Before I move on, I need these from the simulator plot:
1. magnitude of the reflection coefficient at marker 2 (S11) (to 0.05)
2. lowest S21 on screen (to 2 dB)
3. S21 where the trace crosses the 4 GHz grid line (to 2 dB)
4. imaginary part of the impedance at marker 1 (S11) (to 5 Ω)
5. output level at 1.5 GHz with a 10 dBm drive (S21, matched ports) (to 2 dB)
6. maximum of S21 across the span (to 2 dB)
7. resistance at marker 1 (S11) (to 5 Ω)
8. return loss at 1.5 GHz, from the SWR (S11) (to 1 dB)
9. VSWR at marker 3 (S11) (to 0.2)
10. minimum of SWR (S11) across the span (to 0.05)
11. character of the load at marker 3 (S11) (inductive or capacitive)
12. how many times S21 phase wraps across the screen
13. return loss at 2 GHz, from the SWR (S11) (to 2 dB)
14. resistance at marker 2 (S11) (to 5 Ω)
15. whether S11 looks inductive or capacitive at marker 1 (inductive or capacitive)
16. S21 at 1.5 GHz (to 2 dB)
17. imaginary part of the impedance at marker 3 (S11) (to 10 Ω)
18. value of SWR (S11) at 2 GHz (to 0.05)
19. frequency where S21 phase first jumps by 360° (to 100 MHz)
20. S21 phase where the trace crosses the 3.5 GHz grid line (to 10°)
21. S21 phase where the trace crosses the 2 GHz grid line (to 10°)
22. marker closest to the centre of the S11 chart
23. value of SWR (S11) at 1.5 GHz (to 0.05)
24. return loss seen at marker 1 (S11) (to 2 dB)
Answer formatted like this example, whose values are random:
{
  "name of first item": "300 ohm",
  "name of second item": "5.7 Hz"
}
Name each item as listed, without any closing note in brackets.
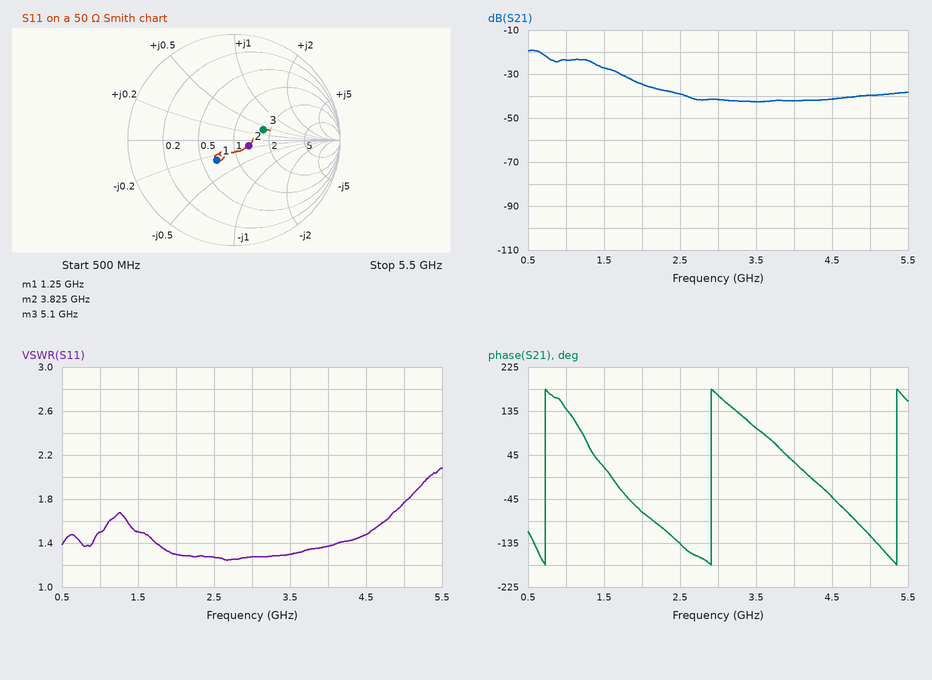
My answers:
{
  "magnitude of the reflection coefficient at marker 2 (S11)": "0.15",
  "lowest S21 on screen": "-42 dB",
  "S21 where the trace crosses the 4 GHz grid line": "-42 dB",
  "imaginary part of the impedance at marker 1 (S11)": "-15 Ω",
  "output level at 1.5 GHz with a 10 dBm drive (S21, matched ports)": "-18 dBm",
  "maximum of S21 across the span": "-20 dB",
  "resistance at marker 1 (S11)": "35 Ω",
  "return loss at 1.5 GHz, from the SWR (S11)": "14 dB",
  "VSWR at marker 3 (S11)": "1.8",
  "minimum of SWR (S11) across the span": "1.25",
  "character of the load at marker 3 (S11)": "inductive",
  "how many times S21 phase wraps across the screen": "3",
  "return loss at 2 GHz, from the SWR (S11)": "18 dB",
  "resistance at marker 2 (S11)": "65 Ω",
  "whether S11 looks inductive or capacitive at marker 1": "capacitive",
  "S21 at 1.5 GHz": "-28 dB",
  "imaginary part of the impedance at marker 3 (S11)": "+20 Ω",
  "value of SWR (S11) at 2 GHz": "1.30",
  "frequency where S21 phase first jumps by 360°": "700 MHz",
  "S21 phase where the trace crosses the 3.5 GHz grid line": "100°",
  "S21 phase where the trace crosses the 2 GHz grid line": "-70°",
  "marker closest to the centre of the S11 chart": "marker 2",
  "value of SWR (S11) at 1.5 GHz": "1.50",
  "return loss seen at marker 1 (S11)": "12 dB"
}
